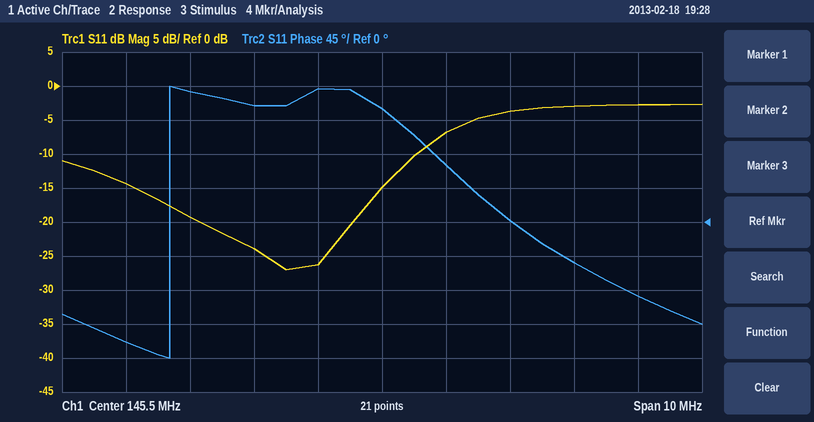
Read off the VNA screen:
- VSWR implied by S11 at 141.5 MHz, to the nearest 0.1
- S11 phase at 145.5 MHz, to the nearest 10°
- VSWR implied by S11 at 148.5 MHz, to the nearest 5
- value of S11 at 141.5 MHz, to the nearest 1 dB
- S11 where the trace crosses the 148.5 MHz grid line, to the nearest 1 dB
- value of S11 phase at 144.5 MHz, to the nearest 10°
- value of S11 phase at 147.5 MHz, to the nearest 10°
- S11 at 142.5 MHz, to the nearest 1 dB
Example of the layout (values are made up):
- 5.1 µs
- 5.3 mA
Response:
- 1.5
- 150°
- 5
- -14 dB
- -3 dB
- 180°
- 0°
- -19 dB
